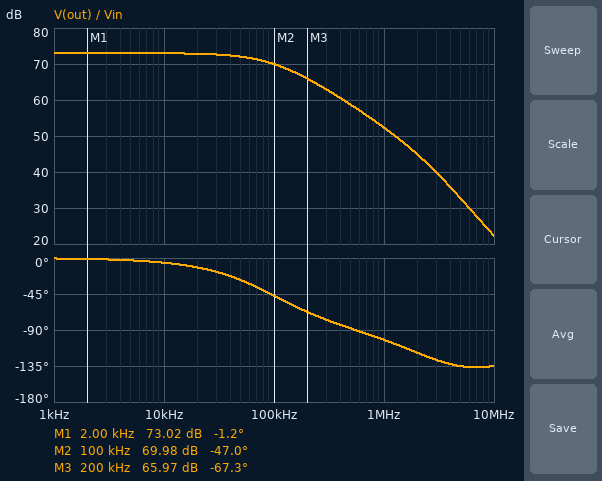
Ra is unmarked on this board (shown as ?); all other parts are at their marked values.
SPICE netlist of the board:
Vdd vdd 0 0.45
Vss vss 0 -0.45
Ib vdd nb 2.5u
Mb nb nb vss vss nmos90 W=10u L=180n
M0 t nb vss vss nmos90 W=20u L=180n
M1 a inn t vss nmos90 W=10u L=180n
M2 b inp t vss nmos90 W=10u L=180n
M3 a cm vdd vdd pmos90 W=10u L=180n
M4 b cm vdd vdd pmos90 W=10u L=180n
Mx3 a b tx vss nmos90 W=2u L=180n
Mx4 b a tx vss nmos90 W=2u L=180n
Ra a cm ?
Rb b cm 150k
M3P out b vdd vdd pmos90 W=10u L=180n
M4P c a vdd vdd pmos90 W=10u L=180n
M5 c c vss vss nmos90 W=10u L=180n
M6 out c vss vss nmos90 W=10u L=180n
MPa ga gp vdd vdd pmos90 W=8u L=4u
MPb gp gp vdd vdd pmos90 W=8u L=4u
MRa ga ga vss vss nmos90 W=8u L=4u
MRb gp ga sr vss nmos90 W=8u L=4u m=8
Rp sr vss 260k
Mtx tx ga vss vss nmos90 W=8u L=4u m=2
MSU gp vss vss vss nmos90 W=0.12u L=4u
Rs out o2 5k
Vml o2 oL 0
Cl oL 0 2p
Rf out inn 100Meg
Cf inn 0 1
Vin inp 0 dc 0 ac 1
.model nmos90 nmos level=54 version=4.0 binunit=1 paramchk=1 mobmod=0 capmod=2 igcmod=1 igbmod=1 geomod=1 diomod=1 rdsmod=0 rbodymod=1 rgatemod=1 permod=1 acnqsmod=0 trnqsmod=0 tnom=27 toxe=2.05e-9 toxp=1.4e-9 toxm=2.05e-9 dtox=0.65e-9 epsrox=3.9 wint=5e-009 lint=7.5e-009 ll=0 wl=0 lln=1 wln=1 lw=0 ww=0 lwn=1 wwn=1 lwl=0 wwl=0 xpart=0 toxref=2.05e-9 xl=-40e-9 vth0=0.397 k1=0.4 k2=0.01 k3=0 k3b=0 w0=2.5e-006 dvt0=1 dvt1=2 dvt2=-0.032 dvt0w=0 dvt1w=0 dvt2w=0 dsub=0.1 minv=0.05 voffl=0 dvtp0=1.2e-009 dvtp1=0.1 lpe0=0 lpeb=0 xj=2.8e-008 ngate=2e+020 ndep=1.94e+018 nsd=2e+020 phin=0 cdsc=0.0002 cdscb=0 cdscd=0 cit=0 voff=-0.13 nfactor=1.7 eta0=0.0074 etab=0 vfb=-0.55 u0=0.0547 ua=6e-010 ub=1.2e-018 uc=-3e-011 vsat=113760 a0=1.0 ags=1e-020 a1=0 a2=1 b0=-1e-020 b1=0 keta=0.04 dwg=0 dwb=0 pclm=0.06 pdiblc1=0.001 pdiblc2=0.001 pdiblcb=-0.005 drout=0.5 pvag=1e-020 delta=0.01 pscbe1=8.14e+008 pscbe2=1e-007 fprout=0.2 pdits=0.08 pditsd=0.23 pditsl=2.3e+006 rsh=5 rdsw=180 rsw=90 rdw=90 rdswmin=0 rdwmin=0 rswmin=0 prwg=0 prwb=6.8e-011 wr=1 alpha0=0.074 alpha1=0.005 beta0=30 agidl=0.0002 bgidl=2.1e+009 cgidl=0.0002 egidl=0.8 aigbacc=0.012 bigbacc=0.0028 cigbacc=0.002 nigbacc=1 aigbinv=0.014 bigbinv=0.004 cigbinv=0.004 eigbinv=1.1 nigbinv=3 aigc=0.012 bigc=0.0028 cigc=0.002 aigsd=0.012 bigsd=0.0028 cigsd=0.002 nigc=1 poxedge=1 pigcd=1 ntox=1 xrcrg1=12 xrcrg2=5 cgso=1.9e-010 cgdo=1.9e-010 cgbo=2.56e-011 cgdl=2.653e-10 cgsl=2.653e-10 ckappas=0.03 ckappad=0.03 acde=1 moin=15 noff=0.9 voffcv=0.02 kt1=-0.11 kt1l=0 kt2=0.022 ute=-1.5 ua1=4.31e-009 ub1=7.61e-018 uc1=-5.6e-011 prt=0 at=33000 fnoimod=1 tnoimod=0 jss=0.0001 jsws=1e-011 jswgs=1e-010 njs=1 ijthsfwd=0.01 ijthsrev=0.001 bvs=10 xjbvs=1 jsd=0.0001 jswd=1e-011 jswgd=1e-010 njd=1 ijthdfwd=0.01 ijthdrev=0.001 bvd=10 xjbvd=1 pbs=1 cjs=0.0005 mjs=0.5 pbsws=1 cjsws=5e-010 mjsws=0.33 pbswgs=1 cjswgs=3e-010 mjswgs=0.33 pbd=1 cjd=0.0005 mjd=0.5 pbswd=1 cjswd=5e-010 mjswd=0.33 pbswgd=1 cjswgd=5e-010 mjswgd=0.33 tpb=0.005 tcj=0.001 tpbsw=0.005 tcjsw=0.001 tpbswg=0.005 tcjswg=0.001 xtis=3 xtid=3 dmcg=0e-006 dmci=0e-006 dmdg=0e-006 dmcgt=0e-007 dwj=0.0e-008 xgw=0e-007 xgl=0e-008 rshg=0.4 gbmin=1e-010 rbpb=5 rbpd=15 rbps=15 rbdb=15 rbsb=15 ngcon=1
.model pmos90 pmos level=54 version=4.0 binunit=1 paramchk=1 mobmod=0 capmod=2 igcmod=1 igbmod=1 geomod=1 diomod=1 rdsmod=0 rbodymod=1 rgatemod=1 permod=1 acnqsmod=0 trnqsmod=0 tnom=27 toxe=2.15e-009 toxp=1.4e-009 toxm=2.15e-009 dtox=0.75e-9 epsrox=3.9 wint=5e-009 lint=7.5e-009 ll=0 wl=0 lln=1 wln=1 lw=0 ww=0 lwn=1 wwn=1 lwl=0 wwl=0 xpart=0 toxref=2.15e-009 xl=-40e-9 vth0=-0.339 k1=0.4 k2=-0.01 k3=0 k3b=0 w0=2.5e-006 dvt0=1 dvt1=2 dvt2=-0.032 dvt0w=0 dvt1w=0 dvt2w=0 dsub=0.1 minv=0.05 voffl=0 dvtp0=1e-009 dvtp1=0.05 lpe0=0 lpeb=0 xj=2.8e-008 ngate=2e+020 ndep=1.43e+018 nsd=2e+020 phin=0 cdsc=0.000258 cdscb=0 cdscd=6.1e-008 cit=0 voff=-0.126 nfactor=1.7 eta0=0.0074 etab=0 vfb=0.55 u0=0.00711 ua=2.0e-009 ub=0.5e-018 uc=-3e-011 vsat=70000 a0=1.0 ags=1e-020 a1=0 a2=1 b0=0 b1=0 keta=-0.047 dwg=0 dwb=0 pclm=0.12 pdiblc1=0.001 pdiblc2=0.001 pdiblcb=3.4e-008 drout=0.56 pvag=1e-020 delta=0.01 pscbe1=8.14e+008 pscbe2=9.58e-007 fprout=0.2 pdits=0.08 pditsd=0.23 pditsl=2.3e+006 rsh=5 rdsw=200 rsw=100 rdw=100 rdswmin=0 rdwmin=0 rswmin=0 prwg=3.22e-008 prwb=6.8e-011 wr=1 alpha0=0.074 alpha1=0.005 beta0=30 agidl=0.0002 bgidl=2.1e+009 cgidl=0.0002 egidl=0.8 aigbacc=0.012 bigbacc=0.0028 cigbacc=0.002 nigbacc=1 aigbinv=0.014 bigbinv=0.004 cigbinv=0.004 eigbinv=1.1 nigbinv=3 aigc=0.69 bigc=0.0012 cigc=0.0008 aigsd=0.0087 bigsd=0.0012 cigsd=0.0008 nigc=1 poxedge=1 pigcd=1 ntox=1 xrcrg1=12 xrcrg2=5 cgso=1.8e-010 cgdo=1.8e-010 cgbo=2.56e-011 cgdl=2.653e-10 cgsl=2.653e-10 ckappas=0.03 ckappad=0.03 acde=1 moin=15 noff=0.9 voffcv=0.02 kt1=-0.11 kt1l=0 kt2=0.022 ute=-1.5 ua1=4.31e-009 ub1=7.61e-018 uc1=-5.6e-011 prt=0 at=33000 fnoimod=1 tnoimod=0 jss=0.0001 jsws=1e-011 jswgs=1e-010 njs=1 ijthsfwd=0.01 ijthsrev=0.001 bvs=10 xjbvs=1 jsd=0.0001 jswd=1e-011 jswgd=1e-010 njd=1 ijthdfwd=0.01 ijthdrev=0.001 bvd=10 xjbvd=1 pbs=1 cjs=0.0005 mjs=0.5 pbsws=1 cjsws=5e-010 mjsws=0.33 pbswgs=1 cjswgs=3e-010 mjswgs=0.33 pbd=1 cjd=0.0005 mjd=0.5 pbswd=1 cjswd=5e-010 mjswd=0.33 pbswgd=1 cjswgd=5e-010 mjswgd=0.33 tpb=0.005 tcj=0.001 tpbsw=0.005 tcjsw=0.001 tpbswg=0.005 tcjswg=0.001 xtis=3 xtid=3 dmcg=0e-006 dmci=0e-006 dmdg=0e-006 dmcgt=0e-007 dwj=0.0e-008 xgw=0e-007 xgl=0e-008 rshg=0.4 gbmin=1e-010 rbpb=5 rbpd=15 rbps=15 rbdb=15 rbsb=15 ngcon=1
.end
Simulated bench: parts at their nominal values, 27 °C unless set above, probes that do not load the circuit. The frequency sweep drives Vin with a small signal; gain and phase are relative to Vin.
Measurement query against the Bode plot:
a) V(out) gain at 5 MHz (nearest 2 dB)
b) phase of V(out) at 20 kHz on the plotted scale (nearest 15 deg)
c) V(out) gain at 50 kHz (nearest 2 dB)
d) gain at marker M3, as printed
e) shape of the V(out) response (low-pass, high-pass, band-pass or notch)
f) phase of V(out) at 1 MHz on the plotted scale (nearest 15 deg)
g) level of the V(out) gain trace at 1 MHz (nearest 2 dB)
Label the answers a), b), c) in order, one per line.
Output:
a) 32 dB
b) -15 deg
c) 72 dB
d) 65.97 dB
e) low-pass
f) -105 deg
g) 52 dB
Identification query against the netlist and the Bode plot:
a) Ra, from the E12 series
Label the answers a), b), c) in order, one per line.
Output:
a) 180 kΩ
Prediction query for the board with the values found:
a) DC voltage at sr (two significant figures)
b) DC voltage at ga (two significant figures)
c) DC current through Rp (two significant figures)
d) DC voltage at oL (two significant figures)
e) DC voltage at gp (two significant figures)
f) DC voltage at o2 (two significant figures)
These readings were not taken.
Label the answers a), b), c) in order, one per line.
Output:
a) -380 mV
b) -150 mV
c) 280 nA
d) 1.6 mV
e) 93 mV
f) 1.6 mV
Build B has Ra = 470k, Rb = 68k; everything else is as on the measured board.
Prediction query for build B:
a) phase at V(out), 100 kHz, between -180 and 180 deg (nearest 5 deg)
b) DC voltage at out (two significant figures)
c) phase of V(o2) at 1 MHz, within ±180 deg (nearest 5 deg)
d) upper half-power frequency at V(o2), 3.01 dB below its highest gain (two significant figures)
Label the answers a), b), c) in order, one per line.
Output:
a) 145 deg
b) 1.8 mV
c) 105 deg
d) 130 kHz
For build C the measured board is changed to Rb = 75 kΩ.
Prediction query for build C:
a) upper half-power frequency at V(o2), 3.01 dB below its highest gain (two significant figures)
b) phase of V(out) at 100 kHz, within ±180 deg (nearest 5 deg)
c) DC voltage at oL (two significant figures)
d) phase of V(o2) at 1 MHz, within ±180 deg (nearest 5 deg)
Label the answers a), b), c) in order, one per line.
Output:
a) 120 kHz
b) -40 deg
c) 1.5 mV
d) -90 deg
